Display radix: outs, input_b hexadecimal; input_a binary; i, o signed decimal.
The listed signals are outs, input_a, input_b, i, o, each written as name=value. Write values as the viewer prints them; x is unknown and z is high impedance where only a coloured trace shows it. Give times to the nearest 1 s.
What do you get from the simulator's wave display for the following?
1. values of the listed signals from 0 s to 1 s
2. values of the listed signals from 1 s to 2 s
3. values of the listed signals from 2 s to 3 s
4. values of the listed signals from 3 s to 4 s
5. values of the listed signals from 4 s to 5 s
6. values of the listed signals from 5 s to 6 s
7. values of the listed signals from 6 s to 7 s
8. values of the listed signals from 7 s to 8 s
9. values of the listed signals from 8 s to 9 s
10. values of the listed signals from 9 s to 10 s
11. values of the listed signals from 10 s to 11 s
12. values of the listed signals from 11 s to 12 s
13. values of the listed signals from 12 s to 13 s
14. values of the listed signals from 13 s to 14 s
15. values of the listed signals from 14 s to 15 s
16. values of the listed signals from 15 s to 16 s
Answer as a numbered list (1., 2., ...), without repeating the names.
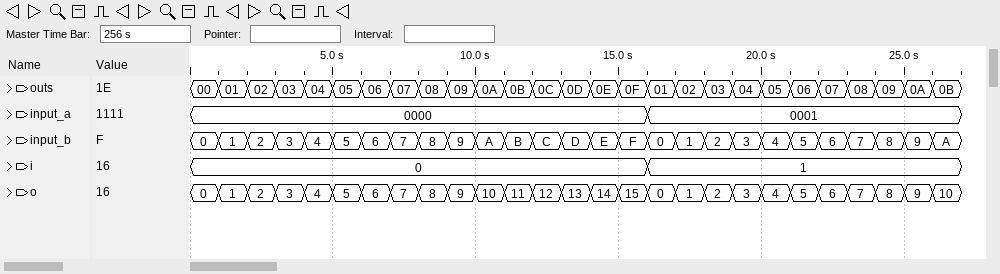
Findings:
1. outs=00, input_a=0000, input_b=0, i=0, o=0
2. outs=01, input_a=0000, input_b=1, i=0, o=1
3. outs=02, input_a=0000, input_b=2, i=0, o=2
4. outs=03, input_a=0000, input_b=3, i=0, o=3
5. outs=04, input_a=0000, input_b=4, i=0, o=4
6. outs=05, input_a=0000, input_b=5, i=0, o=5
7. outs=06, input_a=0000, input_b=6, i=0, o=6
8. outs=07, input_a=0000, input_b=7, i=0, o=7
9. outs=08, input_a=0000, input_b=8, i=0, o=8
10. outs=09, input_a=0000, input_b=9, i=0, o=9
11. outs=0A, input_a=0000, input_b=A, i=0, o=10
12. outs=0B, input_a=0000, input_b=B, i=0, o=11
13. outs=0C, input_a=0000, input_b=C, i=0, o=12
14. outs=0D, input_a=0000, input_b=D, i=0, o=13
15. outs=0E, input_a=0000, input_b=E, i=0, o=14
16. outs=0F, input_a=0000, input_b=F, i=0, o=15
